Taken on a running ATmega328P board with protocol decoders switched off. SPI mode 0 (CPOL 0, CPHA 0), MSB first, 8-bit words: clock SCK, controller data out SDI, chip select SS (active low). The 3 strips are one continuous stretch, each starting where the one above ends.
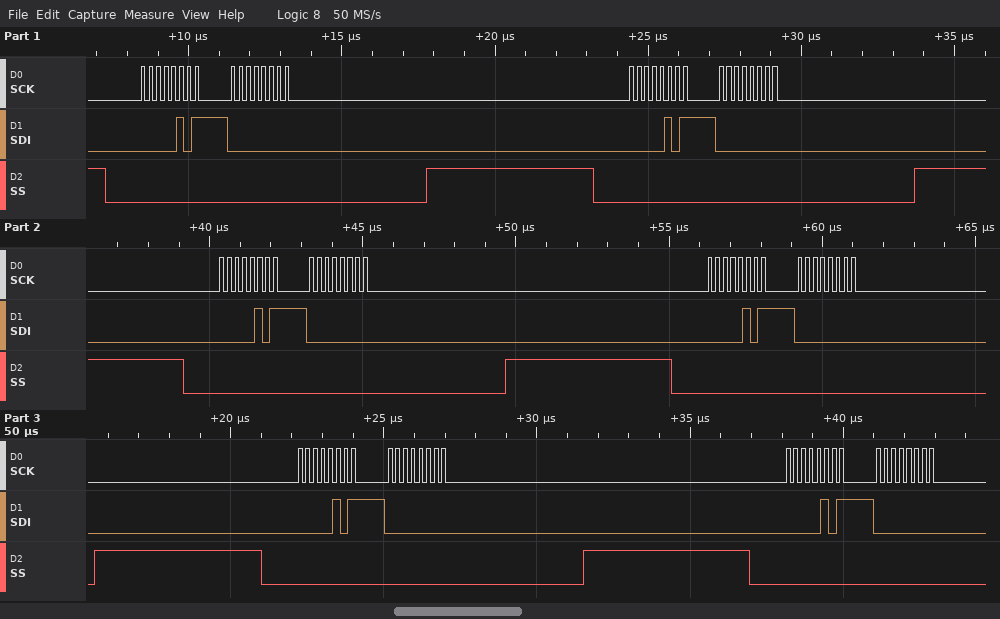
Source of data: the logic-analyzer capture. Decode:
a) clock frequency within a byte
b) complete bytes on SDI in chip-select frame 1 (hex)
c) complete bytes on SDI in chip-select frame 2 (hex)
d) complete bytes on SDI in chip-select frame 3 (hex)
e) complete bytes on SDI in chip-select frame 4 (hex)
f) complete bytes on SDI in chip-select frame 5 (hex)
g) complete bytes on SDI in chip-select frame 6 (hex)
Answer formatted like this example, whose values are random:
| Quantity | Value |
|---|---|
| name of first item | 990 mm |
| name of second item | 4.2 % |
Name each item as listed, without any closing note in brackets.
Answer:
| Quantity | Value |
|---|---|
| clock frequency within a byte | 4 MHz |
| complete bytes on SDI in chip-select frame 1 | 0x05 0x00 |
| complete bytes on SDI in chip-select frame 2 | 0x05 0x00 |
| complete bytes on SDI in chip-select frame 3 | 0x05 0x00 |
| complete bytes on SDI in chip-select frame 4 | 0x05 0x00 |
| complete bytes on SDI in chip-select frame 5 | 0x05 0x00 |
| complete bytes on SDI in chip-select frame 6 | 0x05 0x00 |
